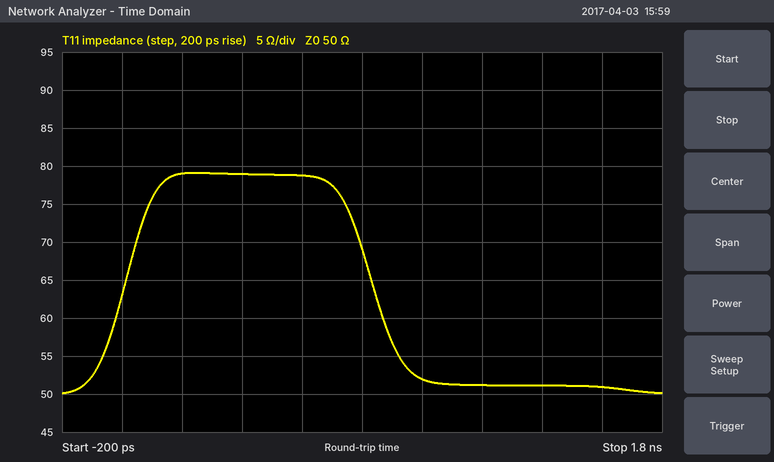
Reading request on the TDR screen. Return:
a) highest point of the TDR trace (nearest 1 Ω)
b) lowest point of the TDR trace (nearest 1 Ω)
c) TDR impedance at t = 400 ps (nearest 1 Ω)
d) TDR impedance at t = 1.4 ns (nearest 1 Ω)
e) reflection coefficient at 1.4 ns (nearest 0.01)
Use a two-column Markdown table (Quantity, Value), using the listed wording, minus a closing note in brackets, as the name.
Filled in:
| Quantity | Value |
|---|---|
| highest point of the TDR trace | 79 Ω |
| lowest point of the TDR trace | 50 Ω |
| TDR impedance at t = 400 ps | 79 Ω |
| TDR impedance at t = 1.4 ns | 51 Ω |
| reflection coefficient at 1.4 ns | +0.01 |
